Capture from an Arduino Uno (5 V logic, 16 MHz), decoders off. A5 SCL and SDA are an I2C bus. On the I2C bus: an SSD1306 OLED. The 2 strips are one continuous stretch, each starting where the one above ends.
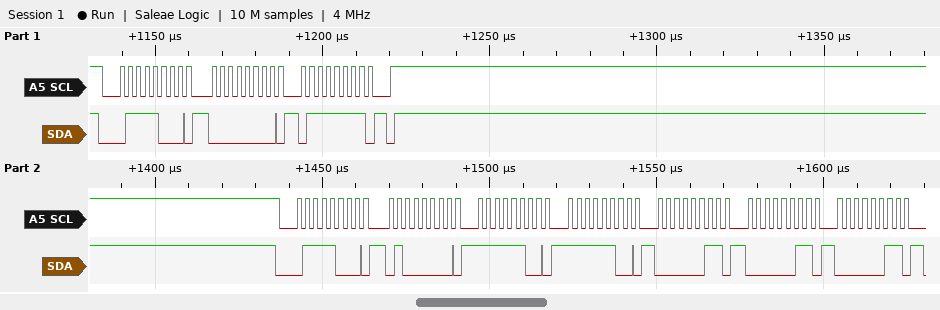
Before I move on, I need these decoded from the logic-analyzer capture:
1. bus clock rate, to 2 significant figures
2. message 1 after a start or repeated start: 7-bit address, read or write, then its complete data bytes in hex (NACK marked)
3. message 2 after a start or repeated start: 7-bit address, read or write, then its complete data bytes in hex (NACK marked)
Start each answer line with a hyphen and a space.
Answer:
- 400 kHz
- 0x3C write: 00 7F
- 0x3C write: 40 FC FC 03 03 03
